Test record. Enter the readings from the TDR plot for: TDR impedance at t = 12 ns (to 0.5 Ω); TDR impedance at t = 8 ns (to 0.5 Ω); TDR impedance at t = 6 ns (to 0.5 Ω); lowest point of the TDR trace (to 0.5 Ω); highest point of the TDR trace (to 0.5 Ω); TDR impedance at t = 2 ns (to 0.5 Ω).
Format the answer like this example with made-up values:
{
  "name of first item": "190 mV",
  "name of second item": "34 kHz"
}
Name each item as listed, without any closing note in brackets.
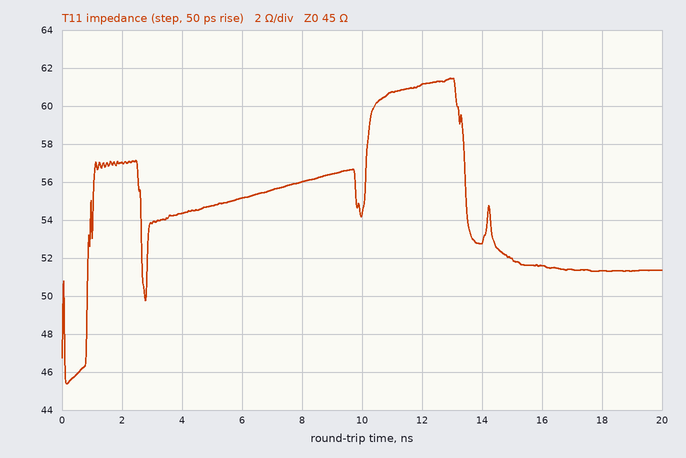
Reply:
{
  "TDR impedance at t = 12 ns": "61.0 Ω",
  "TDR impedance at t = 8 ns": "56.0 Ω",
  "TDR impedance at t = 6 ns": "55.0 Ω",
  "lowest point of the TDR trace": "45.5 Ω",
  "highest point of the TDR trace": "61.5 Ω",
  "TDR impedance at t = 2 ns": "57.0 Ω"
}
